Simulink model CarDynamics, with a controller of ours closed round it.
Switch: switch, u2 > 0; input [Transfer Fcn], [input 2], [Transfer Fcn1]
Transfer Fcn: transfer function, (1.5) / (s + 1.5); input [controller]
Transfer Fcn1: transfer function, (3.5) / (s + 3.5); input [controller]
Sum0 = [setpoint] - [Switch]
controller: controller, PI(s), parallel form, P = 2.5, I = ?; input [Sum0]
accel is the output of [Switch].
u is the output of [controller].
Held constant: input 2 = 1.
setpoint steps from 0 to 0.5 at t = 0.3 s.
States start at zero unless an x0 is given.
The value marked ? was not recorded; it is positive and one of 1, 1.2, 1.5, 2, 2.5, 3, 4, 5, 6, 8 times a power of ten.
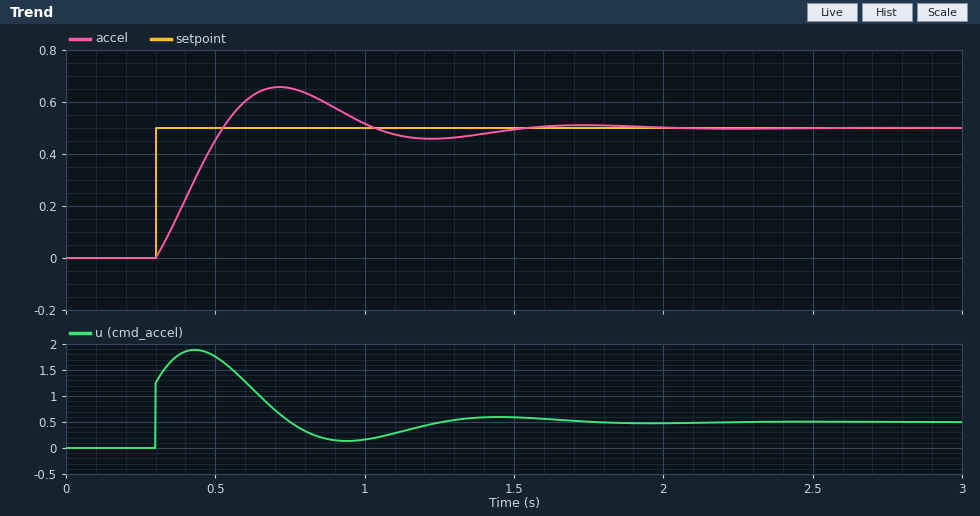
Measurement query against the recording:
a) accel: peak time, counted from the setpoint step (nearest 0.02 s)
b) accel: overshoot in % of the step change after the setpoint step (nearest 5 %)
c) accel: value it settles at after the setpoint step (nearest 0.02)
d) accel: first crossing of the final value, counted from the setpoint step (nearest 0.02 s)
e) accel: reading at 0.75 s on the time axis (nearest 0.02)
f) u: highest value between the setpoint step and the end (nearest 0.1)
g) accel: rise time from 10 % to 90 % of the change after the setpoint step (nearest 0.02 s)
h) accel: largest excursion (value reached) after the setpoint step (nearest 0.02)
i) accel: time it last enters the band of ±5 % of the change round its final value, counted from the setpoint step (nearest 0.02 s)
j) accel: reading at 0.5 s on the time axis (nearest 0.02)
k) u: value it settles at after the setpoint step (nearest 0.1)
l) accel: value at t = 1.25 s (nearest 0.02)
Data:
0.42 s
30 %
0.50
0.22 s
0.66
1.9
0.18 s
0.66
1.08 s
0.46
0.5
0.46
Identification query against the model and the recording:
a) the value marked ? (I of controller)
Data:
30
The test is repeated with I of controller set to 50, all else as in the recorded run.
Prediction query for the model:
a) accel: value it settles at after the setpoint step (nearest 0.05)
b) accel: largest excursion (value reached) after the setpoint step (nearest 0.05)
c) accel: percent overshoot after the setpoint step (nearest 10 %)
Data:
0.50
0.70
40 %
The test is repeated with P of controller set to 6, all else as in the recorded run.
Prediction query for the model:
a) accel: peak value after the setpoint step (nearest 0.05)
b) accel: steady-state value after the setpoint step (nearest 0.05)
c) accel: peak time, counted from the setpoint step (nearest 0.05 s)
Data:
0.55
0.50
0.35 s
